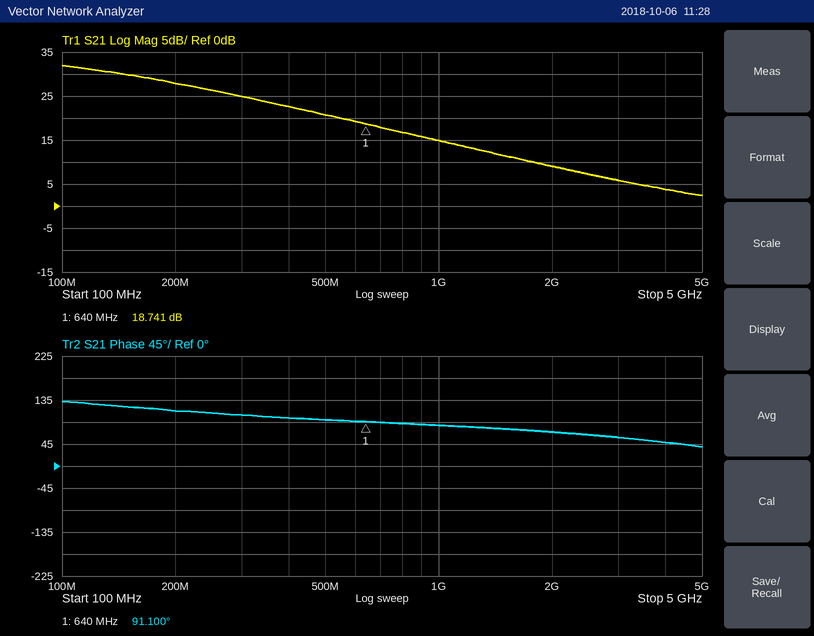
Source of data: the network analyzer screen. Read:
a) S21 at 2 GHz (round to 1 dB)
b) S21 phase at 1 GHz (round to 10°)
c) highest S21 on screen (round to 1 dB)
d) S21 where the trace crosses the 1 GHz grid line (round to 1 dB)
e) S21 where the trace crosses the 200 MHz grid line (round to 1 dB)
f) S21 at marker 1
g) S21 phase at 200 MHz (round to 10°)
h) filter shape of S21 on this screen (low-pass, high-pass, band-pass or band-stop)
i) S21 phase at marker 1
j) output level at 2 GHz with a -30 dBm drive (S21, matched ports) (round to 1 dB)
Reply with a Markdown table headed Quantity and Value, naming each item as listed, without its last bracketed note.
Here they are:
| Quantity | Value |
|---|---|
| S21 at 2 GHz | 9 dB |
| S21 phase at 1 GHz | 80° |
| highest S21 on screen | 32 dB |
| S21 where the trace crosses the 1 GHz grid line | 15 dB |
| S21 where the trace crosses the 200 MHz grid line | 28 dB |
| S21 at marker 1 | 18.741 dB |
| S21 phase at 200 MHz | 110° |
| filter shape of S21 on this screen | low-pass |
| S21 phase at marker 1 | 91.100° |
| output level at 2 GHz with a -30 dBm drive (S21, matched ports) | -21 dBm |
